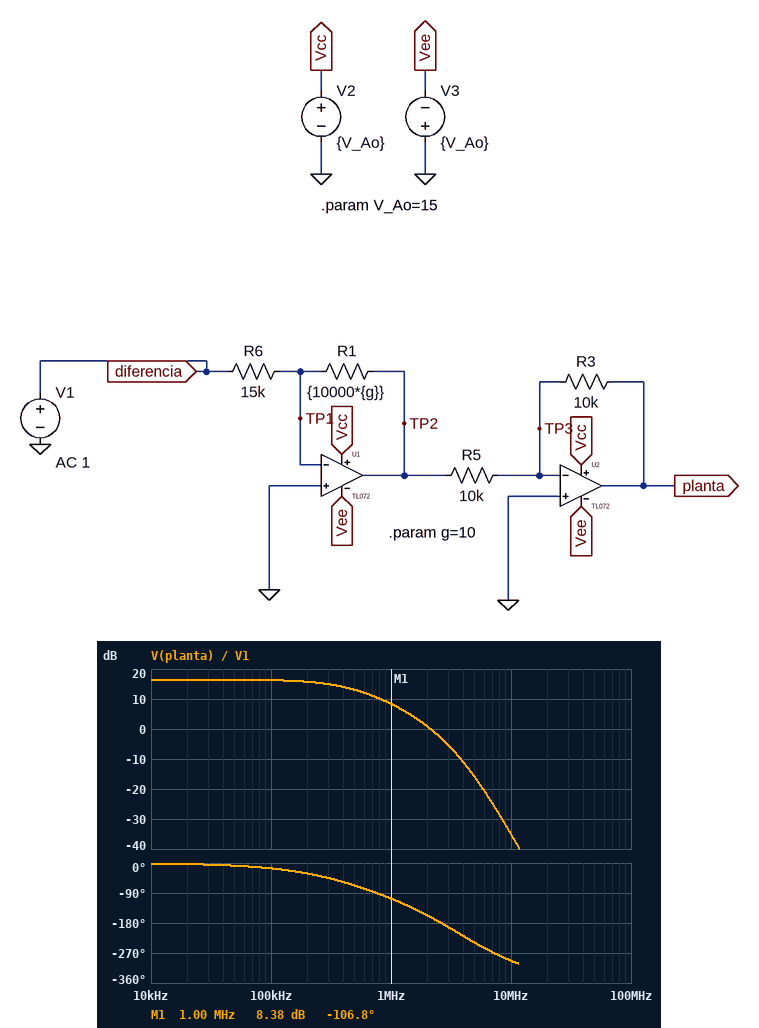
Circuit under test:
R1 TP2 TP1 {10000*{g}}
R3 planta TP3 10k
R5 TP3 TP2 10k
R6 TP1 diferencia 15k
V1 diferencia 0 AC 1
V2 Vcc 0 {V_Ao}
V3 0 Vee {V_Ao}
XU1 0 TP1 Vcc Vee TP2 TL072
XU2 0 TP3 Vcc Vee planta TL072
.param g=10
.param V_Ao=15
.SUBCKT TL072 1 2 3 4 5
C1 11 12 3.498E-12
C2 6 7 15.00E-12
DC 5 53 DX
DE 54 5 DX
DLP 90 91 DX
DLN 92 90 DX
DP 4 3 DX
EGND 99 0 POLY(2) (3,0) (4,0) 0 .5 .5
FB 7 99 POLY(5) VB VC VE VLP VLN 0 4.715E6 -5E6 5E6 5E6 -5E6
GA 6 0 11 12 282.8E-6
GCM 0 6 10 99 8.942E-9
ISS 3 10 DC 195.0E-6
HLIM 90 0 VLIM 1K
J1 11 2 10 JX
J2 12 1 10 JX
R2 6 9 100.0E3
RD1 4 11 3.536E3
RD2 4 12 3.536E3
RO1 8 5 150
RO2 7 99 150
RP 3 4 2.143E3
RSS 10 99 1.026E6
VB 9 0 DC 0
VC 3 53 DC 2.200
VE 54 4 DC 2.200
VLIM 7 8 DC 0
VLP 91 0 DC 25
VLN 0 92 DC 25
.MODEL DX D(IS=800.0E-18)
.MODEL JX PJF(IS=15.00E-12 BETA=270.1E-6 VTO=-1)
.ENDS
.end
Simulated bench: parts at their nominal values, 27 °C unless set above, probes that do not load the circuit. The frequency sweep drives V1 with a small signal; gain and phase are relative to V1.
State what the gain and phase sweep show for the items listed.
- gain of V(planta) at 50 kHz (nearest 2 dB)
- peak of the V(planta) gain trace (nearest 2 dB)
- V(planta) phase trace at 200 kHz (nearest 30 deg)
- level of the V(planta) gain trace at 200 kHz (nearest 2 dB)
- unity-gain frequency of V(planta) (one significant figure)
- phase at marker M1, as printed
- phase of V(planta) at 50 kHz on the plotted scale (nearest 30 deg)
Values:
16 dB
16 dB
-30 deg
16 dB
2 MHz
-106.8 deg
0 deg
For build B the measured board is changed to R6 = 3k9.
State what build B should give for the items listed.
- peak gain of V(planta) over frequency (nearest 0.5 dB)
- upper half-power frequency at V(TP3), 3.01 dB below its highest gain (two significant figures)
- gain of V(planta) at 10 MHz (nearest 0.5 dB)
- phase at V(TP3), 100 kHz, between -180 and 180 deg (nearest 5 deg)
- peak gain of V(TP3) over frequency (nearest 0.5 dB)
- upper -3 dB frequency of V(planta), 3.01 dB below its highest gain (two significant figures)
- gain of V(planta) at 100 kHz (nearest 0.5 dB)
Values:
28.0 dB
2.4 MHz
-34.5 dB
-130 deg
-0.5 dB
130 kHz
26.0 dB
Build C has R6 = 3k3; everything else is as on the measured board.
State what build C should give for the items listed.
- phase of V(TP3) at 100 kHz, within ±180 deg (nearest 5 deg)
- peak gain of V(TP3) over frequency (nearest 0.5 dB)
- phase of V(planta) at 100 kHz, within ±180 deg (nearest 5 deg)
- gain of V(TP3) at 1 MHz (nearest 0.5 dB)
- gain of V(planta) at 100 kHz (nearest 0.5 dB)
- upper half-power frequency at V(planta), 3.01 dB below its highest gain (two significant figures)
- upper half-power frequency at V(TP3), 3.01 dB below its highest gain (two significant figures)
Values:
-135 deg
-0.5 dB
-45 deg
-1.0 dB
27.0 dB
110 kHz
2.4 MHz
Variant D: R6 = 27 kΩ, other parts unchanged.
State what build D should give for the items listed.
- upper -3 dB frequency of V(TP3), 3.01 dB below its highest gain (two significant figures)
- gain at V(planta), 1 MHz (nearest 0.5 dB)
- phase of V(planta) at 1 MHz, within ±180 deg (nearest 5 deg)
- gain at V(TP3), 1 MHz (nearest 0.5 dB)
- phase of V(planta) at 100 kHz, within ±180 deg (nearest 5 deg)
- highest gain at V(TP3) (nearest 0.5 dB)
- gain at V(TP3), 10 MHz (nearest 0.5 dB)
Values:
3.1 MHz
6.5 dB
-95 deg
-4.0 dB
-10 deg
-3.5 dB
-21.5 dB
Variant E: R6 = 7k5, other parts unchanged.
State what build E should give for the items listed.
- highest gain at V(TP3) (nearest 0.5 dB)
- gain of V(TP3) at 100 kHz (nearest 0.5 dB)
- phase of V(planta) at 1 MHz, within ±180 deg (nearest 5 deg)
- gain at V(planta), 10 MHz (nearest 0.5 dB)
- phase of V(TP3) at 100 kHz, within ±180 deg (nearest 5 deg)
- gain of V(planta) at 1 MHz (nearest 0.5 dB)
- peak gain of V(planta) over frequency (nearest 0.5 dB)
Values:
-1.0 dB
-9.0 dB
-120 deg
-34.5 dB
-115 deg
9.5 dB
22.5 dB
